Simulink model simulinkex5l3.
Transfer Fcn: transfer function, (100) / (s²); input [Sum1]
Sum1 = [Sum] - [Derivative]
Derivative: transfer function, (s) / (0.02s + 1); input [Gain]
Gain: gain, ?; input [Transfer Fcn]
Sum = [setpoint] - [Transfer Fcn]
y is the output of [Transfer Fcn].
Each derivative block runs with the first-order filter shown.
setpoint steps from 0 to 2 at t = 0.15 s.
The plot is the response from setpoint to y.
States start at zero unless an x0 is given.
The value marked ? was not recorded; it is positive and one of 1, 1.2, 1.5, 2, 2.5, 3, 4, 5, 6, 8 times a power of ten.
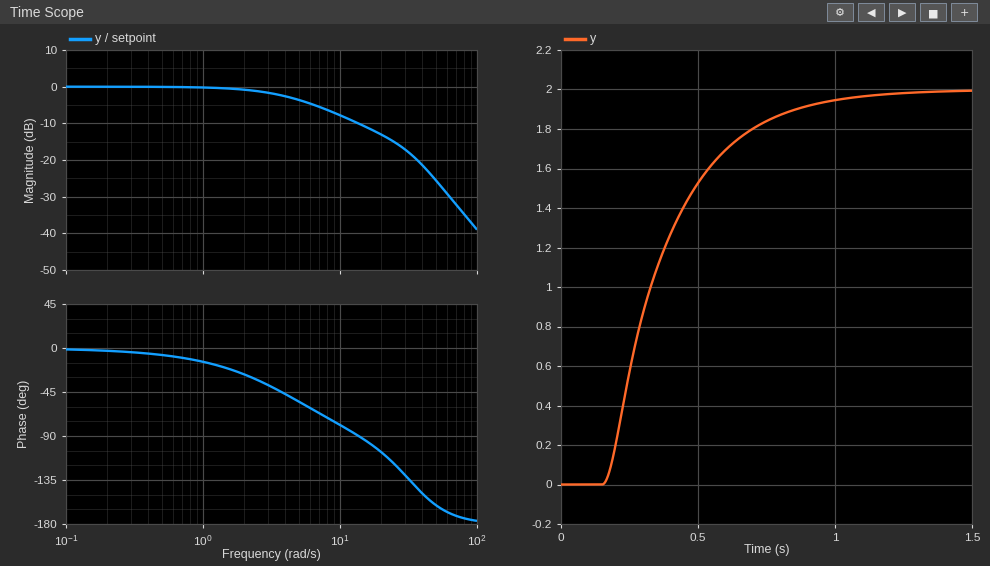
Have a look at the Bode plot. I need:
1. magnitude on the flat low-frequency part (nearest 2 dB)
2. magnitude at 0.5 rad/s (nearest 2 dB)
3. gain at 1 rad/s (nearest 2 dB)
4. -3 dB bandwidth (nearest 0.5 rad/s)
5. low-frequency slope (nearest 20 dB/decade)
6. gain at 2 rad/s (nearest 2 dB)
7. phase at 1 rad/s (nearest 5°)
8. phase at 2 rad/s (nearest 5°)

0 dB
0 dB
0 dB
4.5 rad/s
0 dB/decade
0 dB
-15°
-25°
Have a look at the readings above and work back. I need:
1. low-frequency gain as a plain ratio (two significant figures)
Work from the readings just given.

1.0
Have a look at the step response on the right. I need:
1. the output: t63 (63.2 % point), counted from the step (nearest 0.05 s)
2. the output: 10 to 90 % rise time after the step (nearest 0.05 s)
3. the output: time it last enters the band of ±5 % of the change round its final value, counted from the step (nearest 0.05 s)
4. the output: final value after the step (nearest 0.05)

0.25 s
0.50 s
0.70 s
2.00
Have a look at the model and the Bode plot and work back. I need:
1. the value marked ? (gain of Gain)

0.25
